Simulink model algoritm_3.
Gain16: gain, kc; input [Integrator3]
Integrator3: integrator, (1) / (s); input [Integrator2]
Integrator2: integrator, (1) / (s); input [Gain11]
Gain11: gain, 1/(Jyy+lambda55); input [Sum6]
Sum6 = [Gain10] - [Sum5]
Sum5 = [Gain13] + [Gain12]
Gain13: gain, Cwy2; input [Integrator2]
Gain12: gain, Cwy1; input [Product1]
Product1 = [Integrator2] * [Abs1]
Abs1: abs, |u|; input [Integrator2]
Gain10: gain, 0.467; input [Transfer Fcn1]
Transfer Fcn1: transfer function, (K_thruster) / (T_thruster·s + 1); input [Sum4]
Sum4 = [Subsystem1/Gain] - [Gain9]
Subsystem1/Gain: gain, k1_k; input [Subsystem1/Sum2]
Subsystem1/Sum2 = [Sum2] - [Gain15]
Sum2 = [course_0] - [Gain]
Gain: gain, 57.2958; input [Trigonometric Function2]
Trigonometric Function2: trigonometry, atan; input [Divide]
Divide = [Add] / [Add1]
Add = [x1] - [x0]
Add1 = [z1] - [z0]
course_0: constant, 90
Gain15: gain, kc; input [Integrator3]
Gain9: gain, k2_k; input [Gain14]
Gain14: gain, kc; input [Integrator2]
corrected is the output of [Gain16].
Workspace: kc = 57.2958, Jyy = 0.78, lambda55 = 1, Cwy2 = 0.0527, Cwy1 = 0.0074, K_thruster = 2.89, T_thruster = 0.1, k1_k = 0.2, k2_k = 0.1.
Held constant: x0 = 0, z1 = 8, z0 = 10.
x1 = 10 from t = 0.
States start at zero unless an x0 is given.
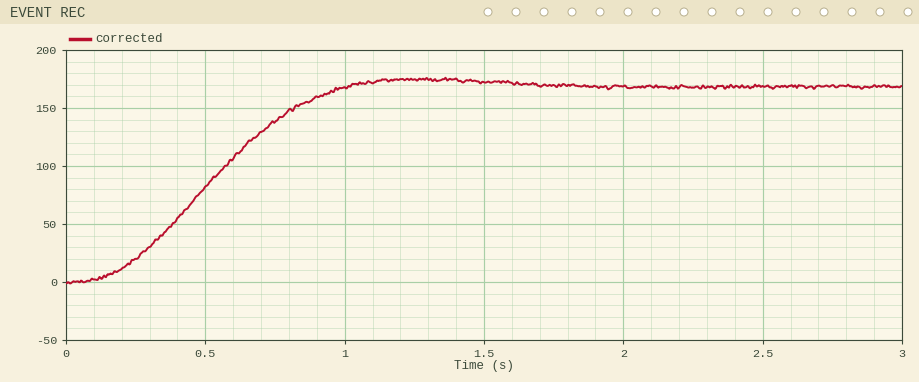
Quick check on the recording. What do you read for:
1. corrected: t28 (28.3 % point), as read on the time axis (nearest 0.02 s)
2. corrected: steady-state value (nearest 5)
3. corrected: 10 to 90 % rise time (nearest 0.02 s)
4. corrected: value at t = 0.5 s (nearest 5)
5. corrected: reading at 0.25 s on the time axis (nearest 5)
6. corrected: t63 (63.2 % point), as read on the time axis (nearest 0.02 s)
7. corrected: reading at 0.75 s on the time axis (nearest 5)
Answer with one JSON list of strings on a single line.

["0.38 s", "170", "0.60 s", "80", "20", "0.60 s", "140"]
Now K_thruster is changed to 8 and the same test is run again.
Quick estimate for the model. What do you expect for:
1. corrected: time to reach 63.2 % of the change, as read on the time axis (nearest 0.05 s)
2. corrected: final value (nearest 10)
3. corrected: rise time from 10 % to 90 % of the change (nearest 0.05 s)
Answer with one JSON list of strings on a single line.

["0.45 s", "170", "0.90 s"]
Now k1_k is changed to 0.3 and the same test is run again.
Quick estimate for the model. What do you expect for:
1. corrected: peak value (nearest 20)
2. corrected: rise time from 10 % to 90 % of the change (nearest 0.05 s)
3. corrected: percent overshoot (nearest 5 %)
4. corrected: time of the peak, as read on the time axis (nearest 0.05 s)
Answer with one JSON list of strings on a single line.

["200", "0.40 s", "20 %", "0.95 s"]
